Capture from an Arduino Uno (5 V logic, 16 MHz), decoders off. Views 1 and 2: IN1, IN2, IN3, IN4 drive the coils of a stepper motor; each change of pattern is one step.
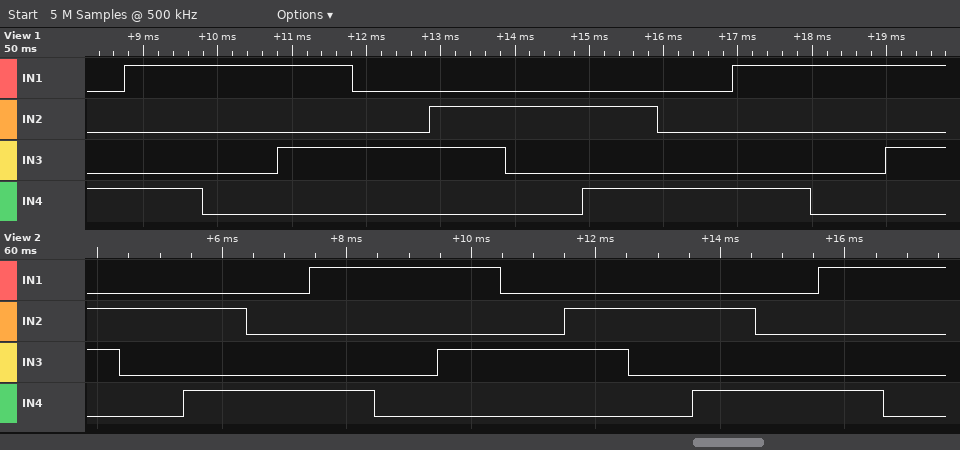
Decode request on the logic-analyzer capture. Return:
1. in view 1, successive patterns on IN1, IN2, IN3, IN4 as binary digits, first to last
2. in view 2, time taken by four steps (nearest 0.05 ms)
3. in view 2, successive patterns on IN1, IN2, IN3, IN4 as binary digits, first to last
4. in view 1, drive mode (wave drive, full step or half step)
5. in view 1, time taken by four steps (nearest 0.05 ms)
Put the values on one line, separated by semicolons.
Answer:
0001 1001 1000 1010 0010 0110 0100 0101 0001 1001 1000 1010; 4.10 ms; 0110 0100 0101 0001 1001 1000 1010 0010 0110 0100 0101 0001 1001 1000; half step; 4.10 ms
